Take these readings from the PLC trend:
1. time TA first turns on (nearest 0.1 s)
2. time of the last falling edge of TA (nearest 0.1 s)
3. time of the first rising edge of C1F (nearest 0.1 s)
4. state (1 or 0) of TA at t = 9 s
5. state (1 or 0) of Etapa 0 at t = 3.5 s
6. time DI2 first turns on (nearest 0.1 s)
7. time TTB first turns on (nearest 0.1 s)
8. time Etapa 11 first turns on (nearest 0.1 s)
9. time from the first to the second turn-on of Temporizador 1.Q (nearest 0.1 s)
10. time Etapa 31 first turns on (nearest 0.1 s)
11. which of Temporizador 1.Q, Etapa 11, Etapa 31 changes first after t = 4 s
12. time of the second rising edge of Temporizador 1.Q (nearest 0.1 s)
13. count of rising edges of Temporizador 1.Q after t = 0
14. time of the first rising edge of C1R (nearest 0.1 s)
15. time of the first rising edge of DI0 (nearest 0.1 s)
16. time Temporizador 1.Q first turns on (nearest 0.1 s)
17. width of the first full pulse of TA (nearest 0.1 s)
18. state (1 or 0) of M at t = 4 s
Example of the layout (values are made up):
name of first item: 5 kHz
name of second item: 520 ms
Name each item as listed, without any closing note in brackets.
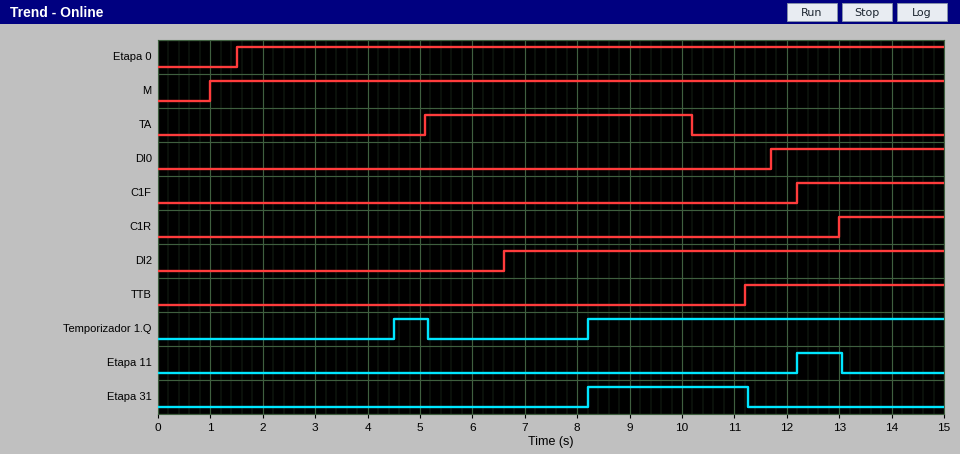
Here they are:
time TA first turns on: 5.1 s
time of the last falling edge of TA: 10.2 s
time of the first rising edge of C1F: 12.2 s
state (1 or 0) of TA at t = 9 s: 1
state (1 or 0) of Etapa 0 at t = 3.5 s: 1
time DI2 first turns on: 6.6 s
time TTB first turns on: 11.2 s
time Etapa 11 first turns on: 12.2 s
time from the first to the second turn-on of Temporizador 1.Q: 3.7 s
time Etapa 31 first turns on: 8.2 s
which of Temporizador 1.Q, Etapa 11, Etapa 31 changes first after t = 4 s: Temporizador 1.Q
time of the second rising edge of Temporizador 1.Q: 8.2 s
count of rising edges of Temporizador 1.Q after t = 0: 2
time of the first rising edge of C1R: 13.0 s
time of the first rising edge of DI0: 11.7 s
time Temporizador 1.Q first turns on: 4.5 s
width of the first full pulse of TA: 5.1 s
state (1 or 0) of M at t = 4 s: 1
